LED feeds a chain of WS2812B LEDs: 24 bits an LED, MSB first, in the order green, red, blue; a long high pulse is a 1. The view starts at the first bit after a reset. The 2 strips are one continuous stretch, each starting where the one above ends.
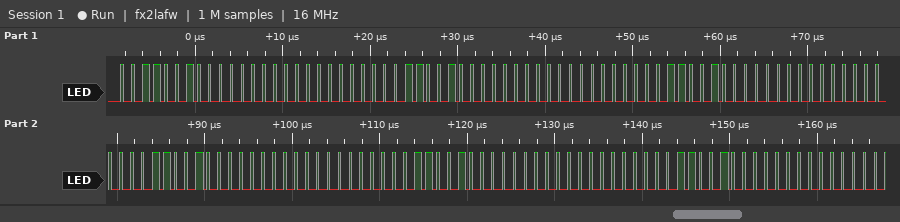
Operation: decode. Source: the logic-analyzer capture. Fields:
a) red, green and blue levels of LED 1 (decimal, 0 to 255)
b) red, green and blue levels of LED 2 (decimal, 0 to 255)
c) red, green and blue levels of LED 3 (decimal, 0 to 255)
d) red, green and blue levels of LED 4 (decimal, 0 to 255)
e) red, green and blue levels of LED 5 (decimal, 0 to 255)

0, 50, 0
0, 50, 0
0, 50, 0
0, 50, 0
0, 50, 0
